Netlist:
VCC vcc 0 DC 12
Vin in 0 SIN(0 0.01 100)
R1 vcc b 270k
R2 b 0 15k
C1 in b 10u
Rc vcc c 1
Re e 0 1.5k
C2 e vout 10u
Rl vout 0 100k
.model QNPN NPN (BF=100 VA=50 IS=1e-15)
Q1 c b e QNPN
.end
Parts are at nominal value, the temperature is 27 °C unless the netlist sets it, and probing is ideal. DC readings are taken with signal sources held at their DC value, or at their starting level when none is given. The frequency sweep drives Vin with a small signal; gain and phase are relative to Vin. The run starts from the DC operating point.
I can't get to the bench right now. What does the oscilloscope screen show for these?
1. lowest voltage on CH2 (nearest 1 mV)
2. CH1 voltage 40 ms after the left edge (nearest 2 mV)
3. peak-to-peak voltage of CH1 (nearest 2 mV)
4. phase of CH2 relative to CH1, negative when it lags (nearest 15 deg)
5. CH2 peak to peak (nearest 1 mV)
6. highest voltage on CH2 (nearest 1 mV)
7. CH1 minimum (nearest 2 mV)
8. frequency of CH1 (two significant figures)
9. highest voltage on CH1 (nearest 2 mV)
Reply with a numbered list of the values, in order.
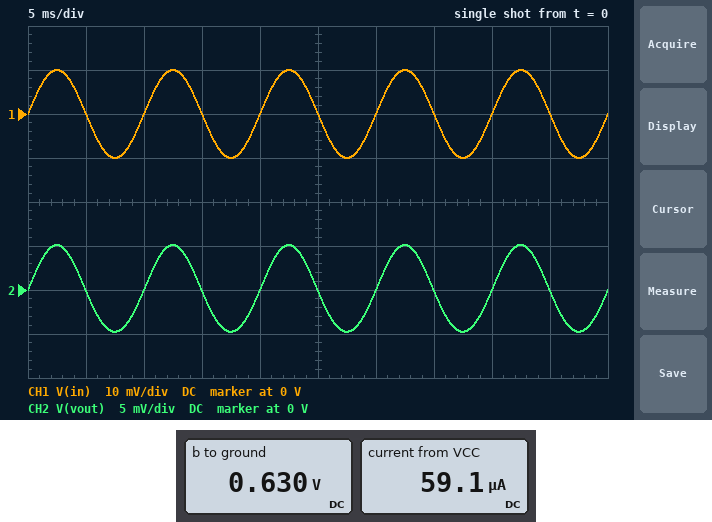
1. -5 mV
2. 0 V
3. 20 mV
4. 0 deg
5. 10 mV
6. 5 mV
7. -10 mV
8. 100 Hz
9. 10 mV
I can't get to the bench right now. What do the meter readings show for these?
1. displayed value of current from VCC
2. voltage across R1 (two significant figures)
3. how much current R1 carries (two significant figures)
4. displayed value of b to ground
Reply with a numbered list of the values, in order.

1. 59.1 µA
2. 11 V
3. 42 µA
4. 0.630 V
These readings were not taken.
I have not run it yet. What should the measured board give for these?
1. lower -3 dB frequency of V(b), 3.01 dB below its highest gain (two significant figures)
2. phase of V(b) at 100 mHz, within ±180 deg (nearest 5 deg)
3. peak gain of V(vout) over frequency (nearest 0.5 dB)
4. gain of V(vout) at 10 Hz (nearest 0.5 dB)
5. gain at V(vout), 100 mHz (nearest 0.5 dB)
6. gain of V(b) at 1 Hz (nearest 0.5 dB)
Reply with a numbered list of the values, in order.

1. 1.2 Hz
2. 85 deg
3. -6.0 dB
4. -6.0 dB
5. -33.0 dB
6. -3.5 dB
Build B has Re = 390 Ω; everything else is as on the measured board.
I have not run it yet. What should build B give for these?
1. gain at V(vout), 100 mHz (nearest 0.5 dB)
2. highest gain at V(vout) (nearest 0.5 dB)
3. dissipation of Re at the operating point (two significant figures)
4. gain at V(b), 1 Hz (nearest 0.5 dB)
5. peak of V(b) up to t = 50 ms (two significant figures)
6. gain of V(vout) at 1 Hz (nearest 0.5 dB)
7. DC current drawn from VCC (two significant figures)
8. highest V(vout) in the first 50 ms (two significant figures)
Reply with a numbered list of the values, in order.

1. -37.5 dB
2. -10.5 dB
3. 320 nW
4. -4.0 dB
5. 640 mV
6. -14.5 dB
7. 70 µA
8. 3.2 mV
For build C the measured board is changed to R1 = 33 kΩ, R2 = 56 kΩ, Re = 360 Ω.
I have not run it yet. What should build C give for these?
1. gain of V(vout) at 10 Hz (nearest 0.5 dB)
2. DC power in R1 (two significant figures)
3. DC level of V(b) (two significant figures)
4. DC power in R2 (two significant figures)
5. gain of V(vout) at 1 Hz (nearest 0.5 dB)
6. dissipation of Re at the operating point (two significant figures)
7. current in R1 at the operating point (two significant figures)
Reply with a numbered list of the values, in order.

1. 0 dB
2. 1.4 mW
3. 5.3 V
4. 500 µW
5. -4.0 dB
6. 56 mW
7. 200 µA
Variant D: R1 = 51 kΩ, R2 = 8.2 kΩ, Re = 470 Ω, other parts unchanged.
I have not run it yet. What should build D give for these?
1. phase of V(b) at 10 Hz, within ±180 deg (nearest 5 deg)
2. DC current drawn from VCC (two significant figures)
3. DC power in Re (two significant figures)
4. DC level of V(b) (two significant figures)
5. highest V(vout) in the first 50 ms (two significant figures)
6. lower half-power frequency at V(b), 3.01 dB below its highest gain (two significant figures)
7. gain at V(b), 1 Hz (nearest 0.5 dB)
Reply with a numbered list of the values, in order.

1. 15 deg
2. 2.0 mA
3. 1.5 mW
4. 1.6 V
5. 9.6 mV
6. 2.5 Hz
7. -8.5 dB
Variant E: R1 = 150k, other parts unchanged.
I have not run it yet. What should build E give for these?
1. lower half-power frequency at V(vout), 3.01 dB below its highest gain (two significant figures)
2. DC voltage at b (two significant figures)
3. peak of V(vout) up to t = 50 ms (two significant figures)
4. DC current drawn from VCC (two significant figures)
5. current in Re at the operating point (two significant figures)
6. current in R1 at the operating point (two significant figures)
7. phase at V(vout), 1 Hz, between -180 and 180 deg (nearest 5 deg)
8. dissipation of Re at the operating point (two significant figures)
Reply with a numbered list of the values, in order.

1. 1.3 Hz
2. 1.1 V
3. 9.3 mV
4. 330 µA
5. 260 µA
6. 73 µA
7. 60 deg
8. 100 µW
